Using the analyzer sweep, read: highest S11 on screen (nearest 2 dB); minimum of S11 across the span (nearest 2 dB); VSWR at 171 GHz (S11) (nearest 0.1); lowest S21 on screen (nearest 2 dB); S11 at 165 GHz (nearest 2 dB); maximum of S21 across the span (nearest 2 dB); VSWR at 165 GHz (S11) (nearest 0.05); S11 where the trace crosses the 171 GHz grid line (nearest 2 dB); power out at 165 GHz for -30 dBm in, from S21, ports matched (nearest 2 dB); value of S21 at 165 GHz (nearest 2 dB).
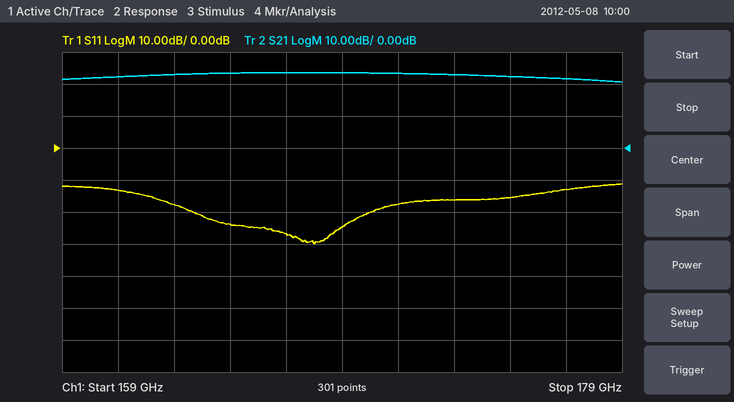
-12 dB
-30 dB
1.3
20 dB
-24 dB
24 dB
1.15
-18 dB
-6 dBm
24 dB
